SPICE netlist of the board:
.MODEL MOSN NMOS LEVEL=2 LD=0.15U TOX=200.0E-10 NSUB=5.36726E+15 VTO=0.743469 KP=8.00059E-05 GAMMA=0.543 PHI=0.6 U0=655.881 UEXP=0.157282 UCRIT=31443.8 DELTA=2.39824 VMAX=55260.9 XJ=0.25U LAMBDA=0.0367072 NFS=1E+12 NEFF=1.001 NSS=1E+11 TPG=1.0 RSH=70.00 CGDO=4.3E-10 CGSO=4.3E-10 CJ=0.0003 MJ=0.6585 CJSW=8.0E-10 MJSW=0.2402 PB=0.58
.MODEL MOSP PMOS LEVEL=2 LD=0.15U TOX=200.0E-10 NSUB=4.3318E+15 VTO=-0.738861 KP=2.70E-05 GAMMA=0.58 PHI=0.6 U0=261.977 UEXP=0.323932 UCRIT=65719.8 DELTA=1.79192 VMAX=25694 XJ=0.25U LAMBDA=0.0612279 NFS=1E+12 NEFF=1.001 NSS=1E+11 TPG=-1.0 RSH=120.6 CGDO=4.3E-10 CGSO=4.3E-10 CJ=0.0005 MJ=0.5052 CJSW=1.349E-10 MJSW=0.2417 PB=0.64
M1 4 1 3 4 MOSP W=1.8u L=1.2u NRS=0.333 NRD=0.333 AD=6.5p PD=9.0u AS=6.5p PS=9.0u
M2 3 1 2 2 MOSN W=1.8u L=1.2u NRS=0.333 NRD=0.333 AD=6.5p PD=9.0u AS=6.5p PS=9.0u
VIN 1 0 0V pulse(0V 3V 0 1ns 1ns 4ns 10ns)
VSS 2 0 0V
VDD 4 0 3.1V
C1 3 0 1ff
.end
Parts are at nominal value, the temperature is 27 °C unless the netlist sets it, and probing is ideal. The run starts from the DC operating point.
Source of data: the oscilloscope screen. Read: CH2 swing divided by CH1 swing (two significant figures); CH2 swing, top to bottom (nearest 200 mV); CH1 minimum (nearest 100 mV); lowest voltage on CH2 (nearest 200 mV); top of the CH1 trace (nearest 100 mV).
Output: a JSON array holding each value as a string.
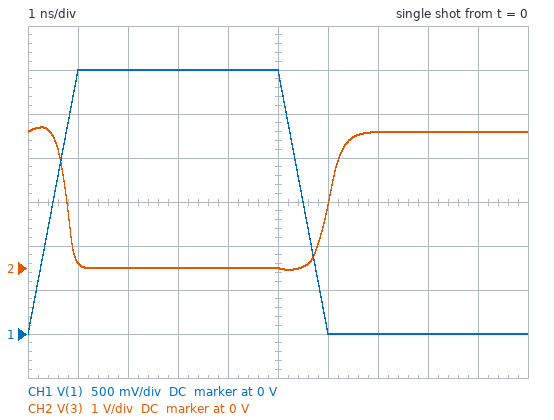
["1.1", "3.2 V", "0 V", "0 V", "3.0 V"]
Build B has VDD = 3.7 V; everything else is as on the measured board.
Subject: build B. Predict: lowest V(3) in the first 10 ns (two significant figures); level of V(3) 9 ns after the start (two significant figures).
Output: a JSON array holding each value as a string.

["-19 mV", "3.7 V"]
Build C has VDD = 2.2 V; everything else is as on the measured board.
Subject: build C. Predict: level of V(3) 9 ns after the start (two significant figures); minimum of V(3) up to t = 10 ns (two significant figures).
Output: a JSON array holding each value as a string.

["2.2 V", "-68 mV"]
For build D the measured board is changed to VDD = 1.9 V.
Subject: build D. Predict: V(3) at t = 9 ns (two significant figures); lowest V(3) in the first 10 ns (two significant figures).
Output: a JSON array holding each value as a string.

["1.9 V", "-92 mV"]
